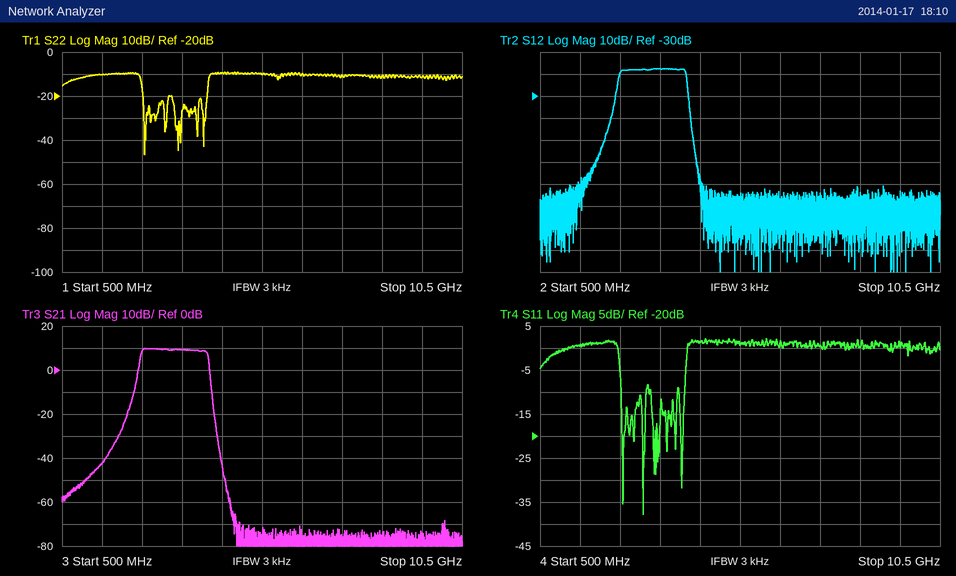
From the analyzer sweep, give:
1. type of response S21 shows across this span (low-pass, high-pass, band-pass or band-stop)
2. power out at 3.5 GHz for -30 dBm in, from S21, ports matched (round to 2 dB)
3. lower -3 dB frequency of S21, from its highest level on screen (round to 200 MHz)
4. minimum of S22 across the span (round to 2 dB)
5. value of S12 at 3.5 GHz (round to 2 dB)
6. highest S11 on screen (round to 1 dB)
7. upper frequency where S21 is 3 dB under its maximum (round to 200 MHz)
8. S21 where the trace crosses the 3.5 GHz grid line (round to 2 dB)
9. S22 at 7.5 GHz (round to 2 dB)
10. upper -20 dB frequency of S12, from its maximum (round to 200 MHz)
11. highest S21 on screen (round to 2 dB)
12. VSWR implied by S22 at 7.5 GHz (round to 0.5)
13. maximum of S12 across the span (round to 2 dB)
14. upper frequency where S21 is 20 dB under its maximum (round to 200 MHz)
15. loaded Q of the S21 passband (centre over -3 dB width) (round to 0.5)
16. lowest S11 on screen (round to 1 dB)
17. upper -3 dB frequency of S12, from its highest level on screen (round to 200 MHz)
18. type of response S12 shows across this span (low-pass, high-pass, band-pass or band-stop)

band-pass
-20 dBm
2.4 GHz
-46 dB
-18 dB
2 dB
4.2 GHz
10 dB
-10 dB
4.2 GHz
10 dB
2.0
-18 dB
4.2 GHz
2.0
-38 dB
4.2 GHz
band-pass
